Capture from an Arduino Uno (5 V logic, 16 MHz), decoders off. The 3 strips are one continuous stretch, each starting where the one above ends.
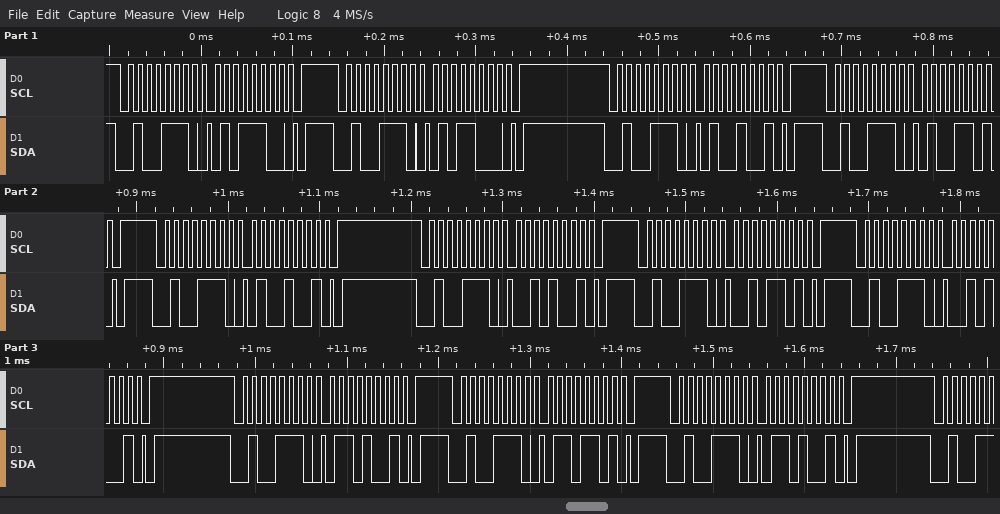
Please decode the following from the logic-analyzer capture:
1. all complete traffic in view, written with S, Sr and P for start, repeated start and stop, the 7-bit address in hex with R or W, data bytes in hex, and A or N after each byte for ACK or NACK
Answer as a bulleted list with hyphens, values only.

- S 27W A 5C A P S 27W A 58 A P S 27W A 49 A P S 27W A 4D A P S 27W A 49 A P S 27W A 29 A P S 27W A 2D A P S 27W A 29 A P S 27W A 69 A P S 27W A 6D A P S 27W A 69 A P
